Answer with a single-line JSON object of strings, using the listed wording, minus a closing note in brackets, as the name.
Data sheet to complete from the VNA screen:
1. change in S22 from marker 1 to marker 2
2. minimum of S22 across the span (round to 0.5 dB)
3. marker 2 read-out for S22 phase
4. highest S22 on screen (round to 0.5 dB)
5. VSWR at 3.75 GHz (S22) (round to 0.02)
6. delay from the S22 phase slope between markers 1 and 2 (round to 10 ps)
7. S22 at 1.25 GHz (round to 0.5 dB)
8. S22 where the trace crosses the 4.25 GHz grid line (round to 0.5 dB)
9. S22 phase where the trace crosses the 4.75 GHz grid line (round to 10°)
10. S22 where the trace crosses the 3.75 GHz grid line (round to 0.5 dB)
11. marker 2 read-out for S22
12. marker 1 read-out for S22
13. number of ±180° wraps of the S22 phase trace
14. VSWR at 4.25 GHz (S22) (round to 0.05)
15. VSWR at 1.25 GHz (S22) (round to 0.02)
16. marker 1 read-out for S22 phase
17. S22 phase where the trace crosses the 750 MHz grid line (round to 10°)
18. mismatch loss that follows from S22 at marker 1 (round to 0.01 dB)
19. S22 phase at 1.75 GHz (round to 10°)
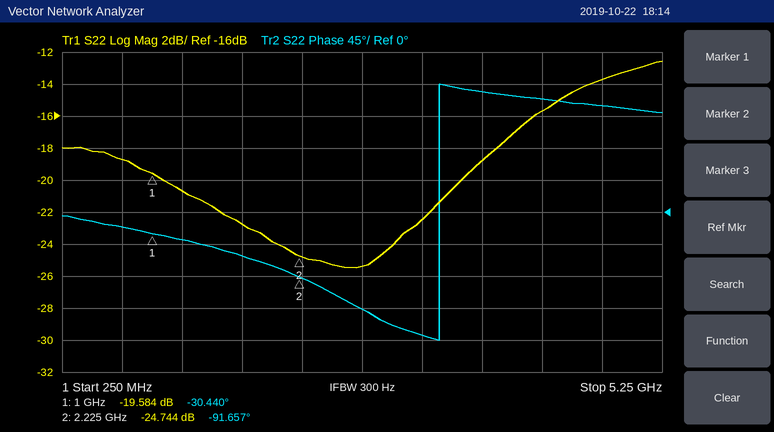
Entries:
{"change in S22 from marker 1 to marker 2": "-5.160 dB", "minimum of S22 across the span": "-25.5 dB", "marker 2 read-out for S22 phase": "-91.657°", "highest S22 on screen": "-12.5 dB", "VSWR at 3.75 GHz (S22)": "1.26", "delay from the S22 phase slope between markers 1 and 2": "140 ps", "S22 at 1.25 GHz": "-20.5 dB", "S22 where the trace crosses the 4.25 GHz grid line": "-15.5 dB", "S22 phase where the trace crosses the 4.75 GHz grid line": "150°", "S22 where the trace crosses the 3.75 GHz grid line": "-19.0 dB", "marker 2 read-out for S22": "-24.744 dB", "marker 1 read-out for S22": "-19.584 dB", "number of ±180° wraps of the S22 phase trace": "1", "VSWR at 4.25 GHz (S22)": "1.40", "VSWR at 1.25 GHz (S22)": "1.20", "marker 1 read-out for S22 phase": "-30.440°", "S22 phase where the trace crosses the 750 MHz grid line": "-20°", "mismatch loss that follows from S22 at marker 1": "0.05 dB", "S22 phase at 1.75 GHz": "-60°"}
